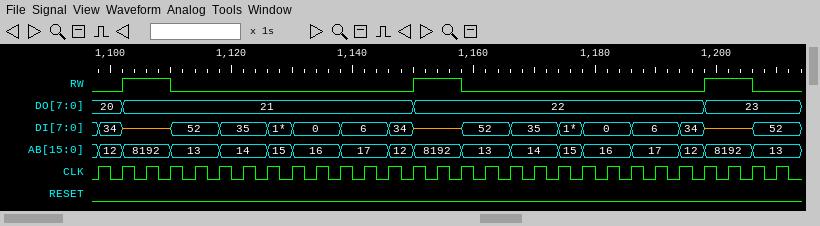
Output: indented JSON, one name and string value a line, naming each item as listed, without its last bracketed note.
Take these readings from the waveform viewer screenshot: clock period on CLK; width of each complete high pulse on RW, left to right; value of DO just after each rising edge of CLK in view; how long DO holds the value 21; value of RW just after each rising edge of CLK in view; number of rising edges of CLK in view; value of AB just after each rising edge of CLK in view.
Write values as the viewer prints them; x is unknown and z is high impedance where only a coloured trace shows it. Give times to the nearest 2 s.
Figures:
{
  "clock period on CLK": "4 s",
  "width of each complete high pulse on RW, left to right": "8 s, 8 s, 8 s",
  "value of DO just after each rising edge of CLK in view": "20, 21, 21, 21, 21, 21, 21, 21, 21, 21, 21, 21, 21, 22, 22, 22, 22, 22, 22, 22, 22, 22, 22, 22, 22, 23, 23, 23, 23",
  "how long DO holds the value 21": "48 s",
  "value of RW just after each rising edge of CLK in view": "0 1 1 0 0 0 0 0 0 0 0 0 0 1 1 0 0 0 0 0 0 0 0 0 0 1 1 0 0",
  "number of rising edges of CLK in view": "29",
  "value of AB just after each rising edge of CLK in view": "12, 8192, 8192, 13, 13, 14, 14, 15, 16, 16, 17, 17, 12, 8192, 8192, 13, 13, 14, 14, 15, 16, 16, 17, 17, 12, 8192, 8192, 13, 13"
}
